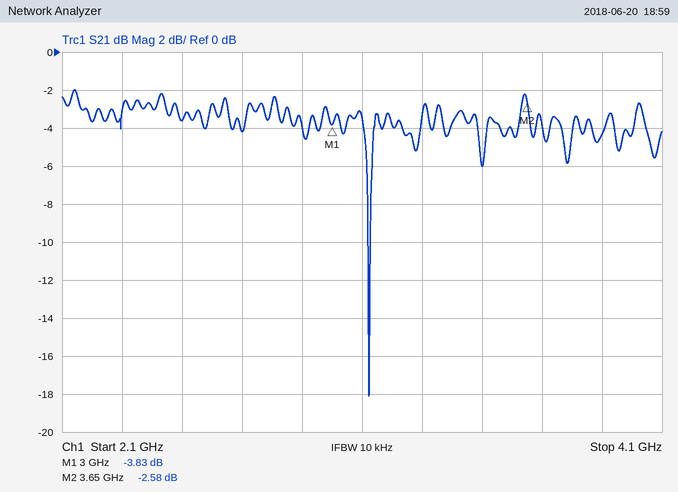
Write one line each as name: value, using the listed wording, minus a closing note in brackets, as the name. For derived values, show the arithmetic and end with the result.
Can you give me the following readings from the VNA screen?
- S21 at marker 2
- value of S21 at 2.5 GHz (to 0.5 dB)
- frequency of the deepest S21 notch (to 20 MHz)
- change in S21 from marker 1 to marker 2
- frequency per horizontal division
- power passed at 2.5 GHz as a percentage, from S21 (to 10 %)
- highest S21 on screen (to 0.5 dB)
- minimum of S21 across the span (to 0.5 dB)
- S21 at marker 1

S21 at marker 2: -2.58 dB
value of S21 at 2.5 GHz: -3.5 dB
frequency of the deepest S21 notch: 3.12 GHz
change in S21 from marker 1 to marker 2: -2.58 − (-3.83) = 1.25 dB
frequency per horizontal division: 200 MHz
power passed at 2.5 GHz as a percentage, from S21: 10^(-3.5/10) ≈ 44.7 %, so 40 % to the nearest 10 %
highest S21 on screen: -2.0 dB
minimum of S21 across the span: -18.0 dB
S21 at marker 1: -3.83 dB
